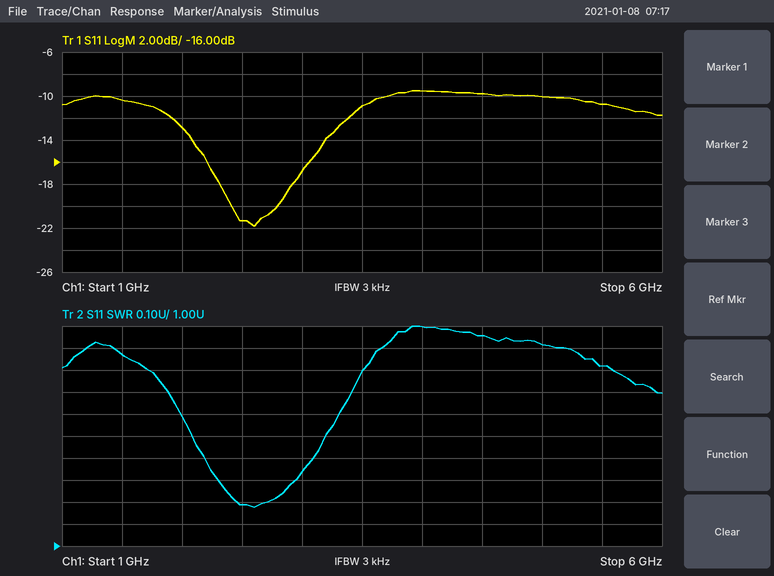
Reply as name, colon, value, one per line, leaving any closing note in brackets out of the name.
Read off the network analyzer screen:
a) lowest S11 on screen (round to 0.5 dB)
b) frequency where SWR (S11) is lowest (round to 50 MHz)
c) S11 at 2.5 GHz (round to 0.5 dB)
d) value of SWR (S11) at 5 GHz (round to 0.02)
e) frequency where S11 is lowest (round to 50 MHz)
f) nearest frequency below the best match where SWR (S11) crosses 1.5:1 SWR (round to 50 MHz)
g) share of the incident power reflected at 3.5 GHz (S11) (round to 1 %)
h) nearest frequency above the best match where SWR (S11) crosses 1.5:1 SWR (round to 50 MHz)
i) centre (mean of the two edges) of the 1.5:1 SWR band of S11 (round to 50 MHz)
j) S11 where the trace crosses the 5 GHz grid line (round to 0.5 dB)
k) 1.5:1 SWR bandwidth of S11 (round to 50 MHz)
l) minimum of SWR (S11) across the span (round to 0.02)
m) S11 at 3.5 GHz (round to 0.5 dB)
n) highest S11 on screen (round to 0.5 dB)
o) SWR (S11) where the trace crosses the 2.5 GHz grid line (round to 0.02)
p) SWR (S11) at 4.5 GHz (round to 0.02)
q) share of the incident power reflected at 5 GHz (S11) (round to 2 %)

lowest S11 on screen: -22.0 dB
frequency where SWR (S11) is lowest: 2.60 GHz
S11 at 2.5 GHz: -21.5 dB
value of SWR (S11) at 5 GHz: 1.92
frequency where S11 is lowest: 2.60 GHz
nearest frequency below the best match where SWR (S11) crosses 1.5:1 SWR: 2.10 GHz
share of the incident power reflected at 3.5 GHz (S11): 8 %
nearest frequency above the best match where SWR (S11) crosses 1.5:1 SWR: 3.20 GHz
centre (mean of the two edges) of the 1.5:1 SWR band of S11: 2.65 GHz
S11 where the trace crosses the 5 GHz grid line: -10.0 dB
1.5:1 SWR bandwidth of S11: 1.10 GHz
minimum of SWR (S11) across the span: 1.18
S11 at 3.5 GHz: -11.0 dB
highest S11 on screen: -9.5 dB
SWR (S11) where the trace crosses the 2.5 GHz grid line: 1.18
SWR (S11) at 4.5 GHz: 1.96
share of the incident power reflected at 5 GHz (S11): 10 %
